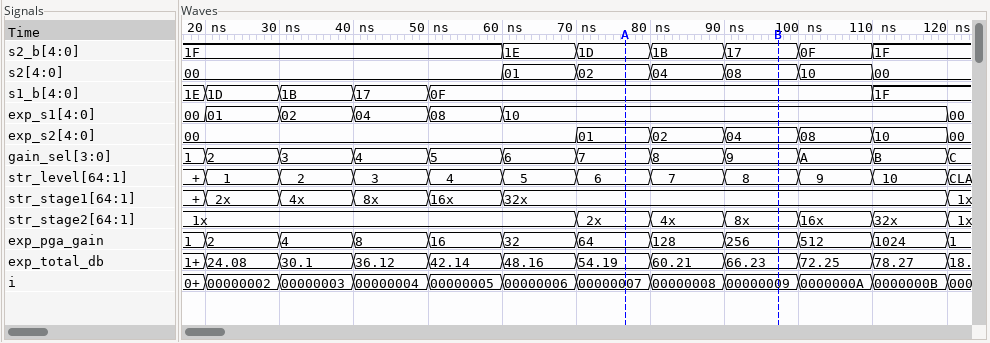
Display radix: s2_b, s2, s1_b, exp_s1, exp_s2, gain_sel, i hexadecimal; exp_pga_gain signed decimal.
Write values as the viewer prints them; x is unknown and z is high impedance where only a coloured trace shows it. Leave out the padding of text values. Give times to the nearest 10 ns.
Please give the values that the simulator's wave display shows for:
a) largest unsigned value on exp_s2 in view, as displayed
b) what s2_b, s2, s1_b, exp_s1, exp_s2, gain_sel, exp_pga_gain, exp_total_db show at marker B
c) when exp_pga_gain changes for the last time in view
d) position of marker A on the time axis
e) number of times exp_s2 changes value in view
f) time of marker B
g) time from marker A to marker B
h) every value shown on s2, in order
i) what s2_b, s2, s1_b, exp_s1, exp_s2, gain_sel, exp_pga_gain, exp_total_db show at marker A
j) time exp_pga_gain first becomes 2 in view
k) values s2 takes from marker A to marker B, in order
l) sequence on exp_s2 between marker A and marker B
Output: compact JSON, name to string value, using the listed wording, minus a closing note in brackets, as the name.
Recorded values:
{"largest unsigned value on exp_s2 in view, as displayed": "10", "what s2_b, s2, s1_b, exp_s1, exp_s2, gain_sel, exp_pga_gain, exp_total_db show at marker B": "s2_b=17, s2=08, s1_b=0F, exp_s1=10, exp_s2=04, gain_sel=9, exp_pga_gain=256, exp_total_db=66.23", "when exp_pga_gain changes for the last time in view": "120 ns", "position of marker A on the time axis": "80 ns", "number of times exp_s2 changes value in view": "6", "time of marker B": "100 ns", "time from marker A to marker B": "20 ns", "every value shown on s2, in order": "00, 01, 02, 04, 08, 10, 00", "what s2_b, s2, s1_b, exp_s1, exp_s2, gain_sel, exp_pga_gain, exp_total_db show at marker A": "s2_b=1D, s2=02, s1_b=0F, exp_s1=10, exp_s2=01, gain_sel=7, exp_pga_gain=64, exp_total_db=54.19", "time exp_pga_gain first becomes 2 in view": "20 ns", "values s2 takes from marker A to marker B, in order": "02, 04, 08", "sequence on exp_s2 between marker A and marker B": "01, 02, 04"}
